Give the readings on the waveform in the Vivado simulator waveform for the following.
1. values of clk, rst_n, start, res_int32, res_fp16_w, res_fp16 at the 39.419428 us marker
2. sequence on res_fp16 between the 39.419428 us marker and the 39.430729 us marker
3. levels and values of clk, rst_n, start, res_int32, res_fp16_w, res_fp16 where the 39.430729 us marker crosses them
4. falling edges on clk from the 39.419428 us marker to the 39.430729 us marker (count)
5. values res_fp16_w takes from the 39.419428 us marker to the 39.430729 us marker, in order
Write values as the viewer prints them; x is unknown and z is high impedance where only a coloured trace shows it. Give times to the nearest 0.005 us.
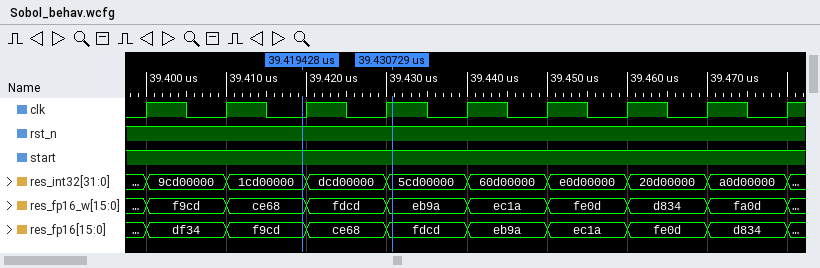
clk=0, rst_n=1, start=1, res_int32=1cd00000, res_fp16_w=ce68, res_fp16=f9cd
f9cd, ce68, fdcd
clk=1, rst_n=1, start=1, res_int32=5cd00000, res_fp16_w=eb9a, res_fp16=fdcd
1
ce68, fdcd, eb9a
